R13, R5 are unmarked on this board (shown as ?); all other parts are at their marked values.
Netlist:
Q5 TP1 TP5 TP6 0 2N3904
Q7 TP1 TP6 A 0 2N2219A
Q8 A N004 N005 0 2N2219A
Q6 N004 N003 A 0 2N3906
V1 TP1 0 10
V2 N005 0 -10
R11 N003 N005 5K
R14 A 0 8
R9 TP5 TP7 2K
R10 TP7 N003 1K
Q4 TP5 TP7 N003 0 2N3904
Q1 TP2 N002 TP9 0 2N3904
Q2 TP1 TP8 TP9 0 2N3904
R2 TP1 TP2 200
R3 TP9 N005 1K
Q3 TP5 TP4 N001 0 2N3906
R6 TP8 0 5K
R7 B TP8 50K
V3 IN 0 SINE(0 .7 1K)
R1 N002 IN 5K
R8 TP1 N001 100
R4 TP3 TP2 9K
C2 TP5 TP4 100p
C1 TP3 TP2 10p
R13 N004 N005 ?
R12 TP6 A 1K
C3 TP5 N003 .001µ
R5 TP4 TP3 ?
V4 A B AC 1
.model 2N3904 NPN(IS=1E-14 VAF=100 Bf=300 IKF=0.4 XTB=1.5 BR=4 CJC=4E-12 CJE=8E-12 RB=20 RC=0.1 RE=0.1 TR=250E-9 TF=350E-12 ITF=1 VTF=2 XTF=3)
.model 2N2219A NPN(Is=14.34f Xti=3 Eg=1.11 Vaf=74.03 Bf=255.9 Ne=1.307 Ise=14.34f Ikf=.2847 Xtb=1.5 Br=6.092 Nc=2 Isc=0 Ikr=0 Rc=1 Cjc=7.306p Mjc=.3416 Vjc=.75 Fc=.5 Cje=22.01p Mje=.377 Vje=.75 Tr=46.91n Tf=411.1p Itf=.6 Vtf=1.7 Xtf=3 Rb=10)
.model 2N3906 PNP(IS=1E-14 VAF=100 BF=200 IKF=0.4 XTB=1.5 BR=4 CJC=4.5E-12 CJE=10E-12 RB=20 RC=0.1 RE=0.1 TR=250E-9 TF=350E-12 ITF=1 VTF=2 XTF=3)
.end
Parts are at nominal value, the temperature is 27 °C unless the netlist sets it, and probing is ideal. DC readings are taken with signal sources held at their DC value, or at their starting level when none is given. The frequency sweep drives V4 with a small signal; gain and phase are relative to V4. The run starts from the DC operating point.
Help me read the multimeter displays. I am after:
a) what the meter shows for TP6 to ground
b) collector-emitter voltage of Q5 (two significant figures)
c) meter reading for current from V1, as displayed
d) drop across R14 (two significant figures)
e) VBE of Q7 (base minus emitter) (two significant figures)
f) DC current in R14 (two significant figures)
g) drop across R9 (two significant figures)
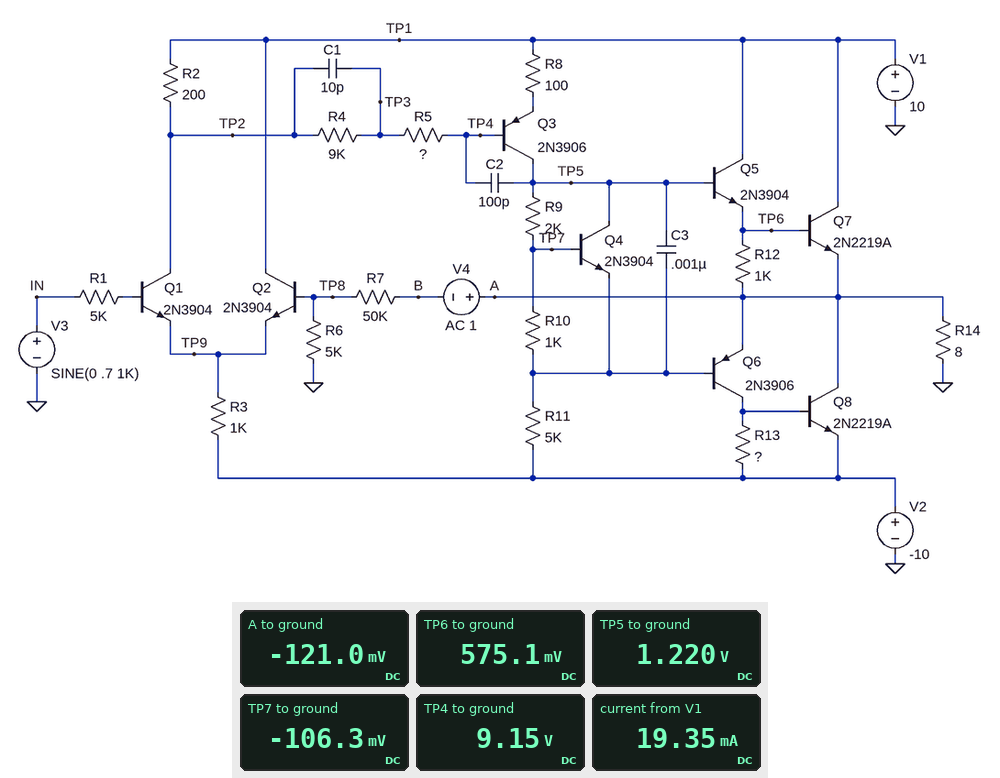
575.1 mV
9.4 V
19.35 mA
120 mV
700 mV
15 mA
1.3 V
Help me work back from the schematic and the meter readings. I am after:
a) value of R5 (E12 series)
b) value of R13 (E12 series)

560 Ω
1.2 kΩ
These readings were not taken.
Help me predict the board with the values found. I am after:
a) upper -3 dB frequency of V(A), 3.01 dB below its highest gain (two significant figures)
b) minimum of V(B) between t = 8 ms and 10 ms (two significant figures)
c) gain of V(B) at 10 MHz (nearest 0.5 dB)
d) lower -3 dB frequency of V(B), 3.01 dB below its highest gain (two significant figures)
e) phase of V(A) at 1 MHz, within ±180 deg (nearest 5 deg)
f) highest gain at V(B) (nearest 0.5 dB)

71 kHz
-7.3 V
0 dB
69 kHz
-105 deg
0 dB
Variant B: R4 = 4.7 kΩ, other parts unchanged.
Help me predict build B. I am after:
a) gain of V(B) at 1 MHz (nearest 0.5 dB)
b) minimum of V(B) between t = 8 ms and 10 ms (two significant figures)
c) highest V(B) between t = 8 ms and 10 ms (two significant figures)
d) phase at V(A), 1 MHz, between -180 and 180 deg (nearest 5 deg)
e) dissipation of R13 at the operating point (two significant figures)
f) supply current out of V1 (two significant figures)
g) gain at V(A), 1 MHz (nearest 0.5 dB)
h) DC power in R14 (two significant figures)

0.5 dB
-7.3 V
7.3 V
-120 deg
420 µW
20 mA
-20.5 dB
210 µW
